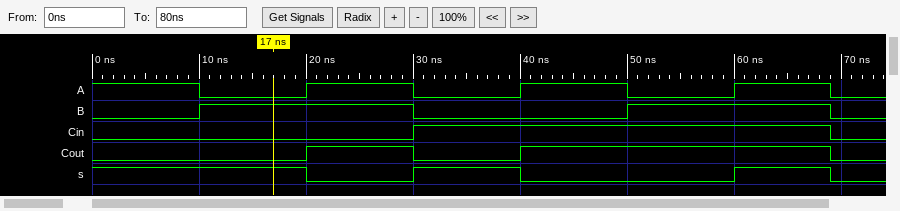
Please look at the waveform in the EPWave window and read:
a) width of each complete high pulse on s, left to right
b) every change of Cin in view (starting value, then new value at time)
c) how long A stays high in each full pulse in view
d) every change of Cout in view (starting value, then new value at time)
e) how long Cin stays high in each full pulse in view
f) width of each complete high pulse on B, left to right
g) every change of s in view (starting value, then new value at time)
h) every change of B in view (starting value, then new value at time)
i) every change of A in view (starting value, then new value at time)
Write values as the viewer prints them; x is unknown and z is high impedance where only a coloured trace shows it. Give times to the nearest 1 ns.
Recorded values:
10 ns, 9 ns
0, 1 at 30 ns, 0 at 69 ns
10 ns, 10 ns, 9 ns
0, 1 at 20 ns, 0 at 30 ns, 1 at 40 ns, 0 at 69 ns
39 ns
20 ns, 19 ns
1, 0 at 20 ns, 1 at 30 ns, 0 at 40 ns, 1 at 60 ns, 0 at 69 ns
0, 1 at 10 ns, 0 at 30 ns, 1 at 50 ns, 0 at 69 ns
1, 0 at 10 ns, 1 at 20 ns, 0 at 30 ns, 1 at 40 ns, 0 at 50 ns, 1 at 60 ns, 0 at 69 ns
